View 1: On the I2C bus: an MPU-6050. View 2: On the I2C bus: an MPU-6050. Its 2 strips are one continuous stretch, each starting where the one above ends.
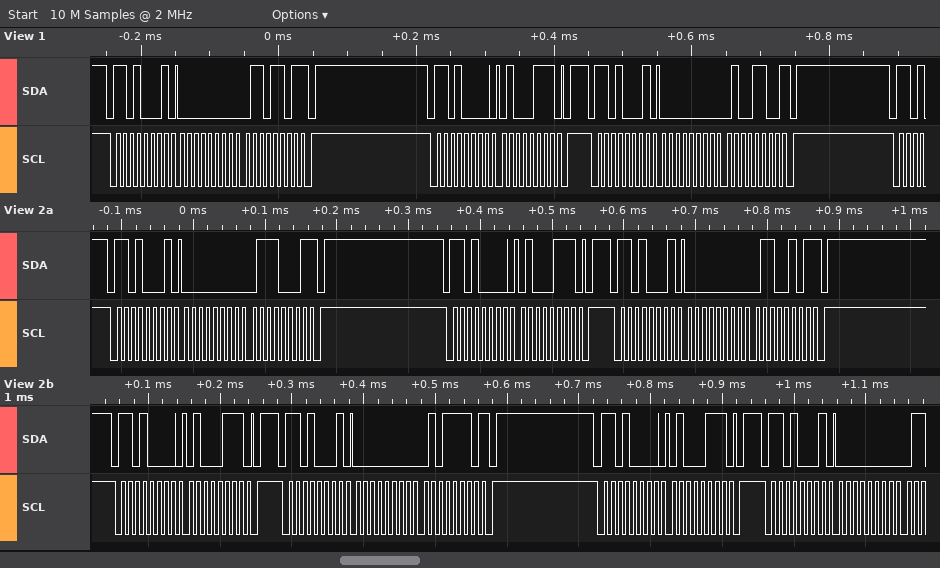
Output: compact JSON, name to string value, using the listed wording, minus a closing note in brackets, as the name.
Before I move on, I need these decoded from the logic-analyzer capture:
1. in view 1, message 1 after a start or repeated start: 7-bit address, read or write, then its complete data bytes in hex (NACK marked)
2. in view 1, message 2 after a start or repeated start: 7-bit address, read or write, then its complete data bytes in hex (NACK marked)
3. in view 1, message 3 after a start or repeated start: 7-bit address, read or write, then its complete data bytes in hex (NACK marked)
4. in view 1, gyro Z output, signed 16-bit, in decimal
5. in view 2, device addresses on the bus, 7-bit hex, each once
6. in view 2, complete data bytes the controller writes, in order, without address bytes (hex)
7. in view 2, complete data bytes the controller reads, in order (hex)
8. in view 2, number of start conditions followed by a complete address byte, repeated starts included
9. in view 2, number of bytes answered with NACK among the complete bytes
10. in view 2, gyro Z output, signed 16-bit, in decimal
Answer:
{"in view 1, message 1 after a start or repeated start: 7-bit address, read or write, then its complete data bytes in hex": "0x68 read: 00 6D NACK", "in view 1, message 2 after a start or repeated start: 7-bit address, read or write, then its complete data bytes in hex": "0x68 write: 47", "in view 1, message 3 after a start or repeated start: 7-bit address, read or write, then its complete data bytes in hex": "0x68 read: 00 4C NACK", "in view 1, gyro Z output, signed 16-bit, in decimal": "76", "in view 2, device addresses on the bus, 7-bit hex, each once": "0x68", "in view 2, complete data bytes the controller writes, in order, without address bytes": "47 47 47", "in view 2, complete data bytes the controller reads, in order": "00 71 00 65 00 5E 00", "in view 2, number of start conditions followed by a complete address byte, repeated starts included": "7", "in view 2, number of bytes answered with NACK among the complete bytes": "3", "in view 2, gyro Z output, signed 16-bit, in decimal": "101"}
